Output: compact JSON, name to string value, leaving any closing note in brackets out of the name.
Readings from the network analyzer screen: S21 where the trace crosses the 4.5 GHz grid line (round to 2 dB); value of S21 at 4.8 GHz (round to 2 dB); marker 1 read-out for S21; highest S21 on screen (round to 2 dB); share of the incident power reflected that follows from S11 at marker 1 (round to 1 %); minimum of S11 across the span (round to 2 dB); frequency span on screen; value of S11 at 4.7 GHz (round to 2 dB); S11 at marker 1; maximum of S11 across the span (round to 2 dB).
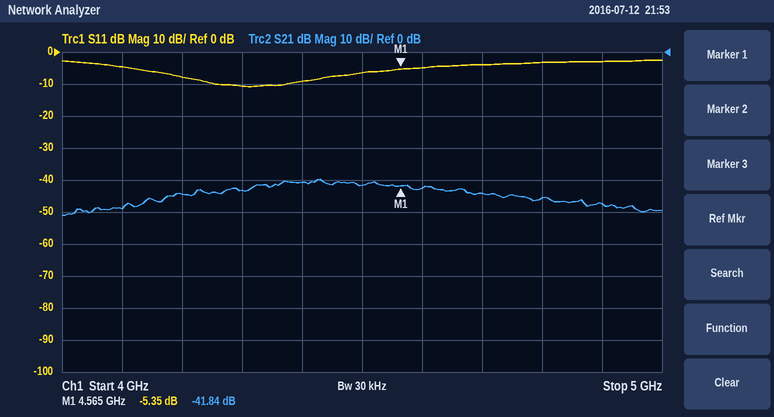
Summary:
{"S21 where the trace crosses the 4.5 GHz grid line": "-42 dB", "value of S21 at 4.8 GHz": "-46 dB", "marker 1 read-out for S21": "-41.84 dB", "highest S21 on screen": "-40 dB", "share of the incident power reflected that follows from S11 at marker 1": "29 %", "minimum of S11 across the span": "-10 dB", "frequency span on screen": "1 GHz", "value of S11 at 4.7 GHz": "-4 dB", "S11 at marker 1": "-5.35 dB", "maximum of S11 across the span": "-2 dB"}
